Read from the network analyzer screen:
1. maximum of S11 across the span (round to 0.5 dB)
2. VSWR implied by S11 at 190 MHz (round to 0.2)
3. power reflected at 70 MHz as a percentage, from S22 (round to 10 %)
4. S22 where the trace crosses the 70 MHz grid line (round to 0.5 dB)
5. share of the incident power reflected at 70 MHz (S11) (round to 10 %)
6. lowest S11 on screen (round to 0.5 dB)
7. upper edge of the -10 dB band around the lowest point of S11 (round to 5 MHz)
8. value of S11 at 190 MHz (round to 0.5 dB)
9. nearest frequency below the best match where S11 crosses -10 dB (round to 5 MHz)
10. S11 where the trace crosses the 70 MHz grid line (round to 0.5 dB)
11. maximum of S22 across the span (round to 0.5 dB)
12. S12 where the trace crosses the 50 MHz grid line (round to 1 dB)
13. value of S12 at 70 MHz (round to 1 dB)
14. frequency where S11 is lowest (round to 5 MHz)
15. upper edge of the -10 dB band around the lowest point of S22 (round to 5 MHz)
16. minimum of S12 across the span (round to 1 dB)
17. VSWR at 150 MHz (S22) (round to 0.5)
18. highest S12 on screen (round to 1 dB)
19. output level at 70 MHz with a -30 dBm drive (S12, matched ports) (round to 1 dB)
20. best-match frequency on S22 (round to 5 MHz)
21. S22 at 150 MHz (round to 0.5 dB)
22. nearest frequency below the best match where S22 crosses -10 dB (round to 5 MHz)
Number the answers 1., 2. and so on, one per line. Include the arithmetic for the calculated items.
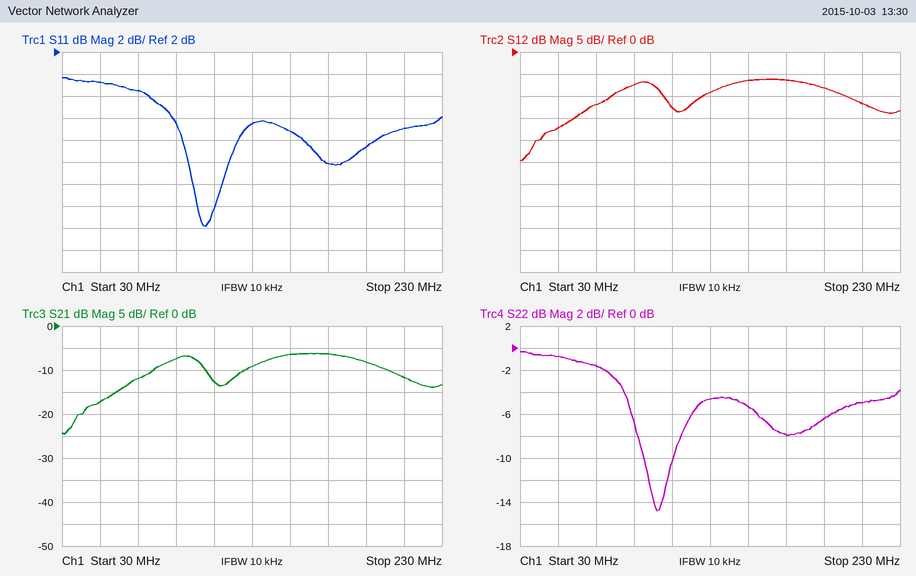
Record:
1. -0.5 dB
2. |Γ| = 10^(-6.5/20) = 0.4732; VSWR = (1 + 0.4732)/(1 − 0.4732) ≈ 2.8
3. 10^(-1.5/10) ≈ 70.8 %, so 70 % to the nearest 10 %
4. -1.5 dB
5. 10^(-1.5/10) ≈ 70.8 %, so 70 % to the nearest 10 %
6. -14.0 dB
7. 115 MHz
8. -6.5 dB
9. 100 MHz
10. -1.5 dB
11. -0.5 dB
12. -17 dB
13. -12 dB
14. 105 MHz
15. 110 MHz
16. -25 dB
17. |Γ| = 10^(-5.5/20) = 0.5309; VSWR = (1 + 0.5309)/(1 − 0.5309) ≈ 3.26, so 3.5 to the nearest 0.5
18. -6 dB
19. -30 dBm + (-12 dB) = -42 dBm
20. 100 MHz
21. -5.5 dB
22. 95 MHz
